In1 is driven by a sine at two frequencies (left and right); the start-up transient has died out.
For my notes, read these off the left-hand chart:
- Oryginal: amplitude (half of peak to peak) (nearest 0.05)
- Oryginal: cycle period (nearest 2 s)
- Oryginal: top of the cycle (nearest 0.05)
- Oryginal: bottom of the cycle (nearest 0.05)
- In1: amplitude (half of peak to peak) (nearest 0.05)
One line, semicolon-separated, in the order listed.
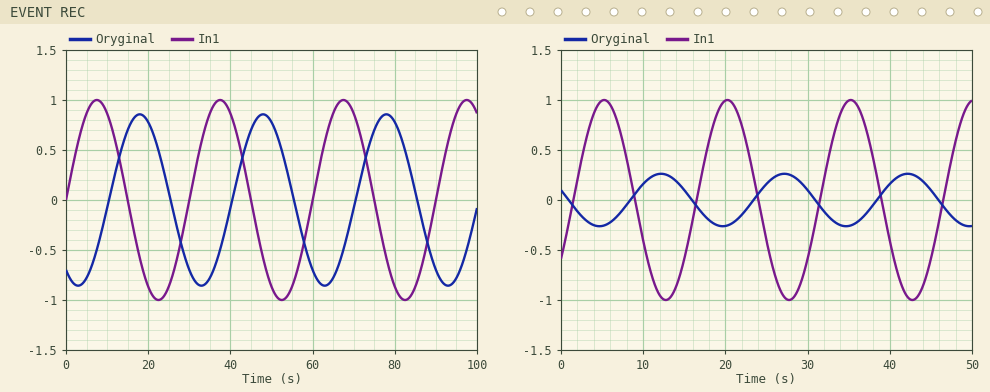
0.85; 30 s; 0.85; -0.85; 1.00
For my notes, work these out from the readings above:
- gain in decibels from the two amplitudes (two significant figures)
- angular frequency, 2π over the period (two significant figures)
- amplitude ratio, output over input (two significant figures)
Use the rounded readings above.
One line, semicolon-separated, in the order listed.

-1.4 dB; 0.21 rad/s; 0.85
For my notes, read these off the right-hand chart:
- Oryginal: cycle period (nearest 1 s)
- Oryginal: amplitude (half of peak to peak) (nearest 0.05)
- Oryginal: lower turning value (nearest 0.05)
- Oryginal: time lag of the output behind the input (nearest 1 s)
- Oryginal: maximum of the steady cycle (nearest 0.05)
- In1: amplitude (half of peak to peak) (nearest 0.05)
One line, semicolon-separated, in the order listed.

15 s; 0.25; -0.25; 7 s; 0.25; 1.00
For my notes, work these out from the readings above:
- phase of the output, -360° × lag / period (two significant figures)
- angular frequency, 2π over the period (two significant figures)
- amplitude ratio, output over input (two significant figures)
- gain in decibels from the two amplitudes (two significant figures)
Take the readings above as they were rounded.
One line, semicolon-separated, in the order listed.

-170°; 0.42 rad/s; 0.25; -12 dB
